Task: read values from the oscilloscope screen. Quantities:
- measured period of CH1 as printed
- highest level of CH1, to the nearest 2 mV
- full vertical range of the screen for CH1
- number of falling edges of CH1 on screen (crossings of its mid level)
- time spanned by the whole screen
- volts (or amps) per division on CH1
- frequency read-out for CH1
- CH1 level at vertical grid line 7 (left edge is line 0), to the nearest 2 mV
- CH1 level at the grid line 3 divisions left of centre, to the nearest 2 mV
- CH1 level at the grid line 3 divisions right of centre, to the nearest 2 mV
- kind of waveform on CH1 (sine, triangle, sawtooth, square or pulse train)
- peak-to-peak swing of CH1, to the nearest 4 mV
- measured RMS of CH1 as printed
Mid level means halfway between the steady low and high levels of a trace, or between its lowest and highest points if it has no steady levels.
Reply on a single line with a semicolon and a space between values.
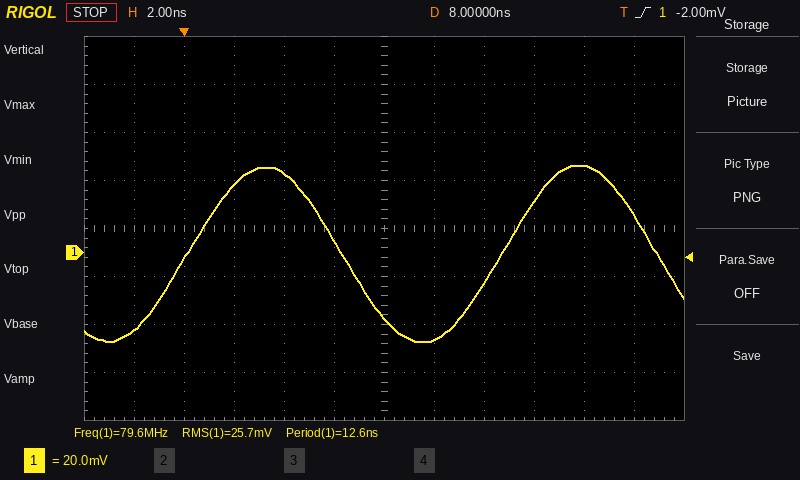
12.6 ns; 36 mV; 160 mV; 2; 24 ns; 20 mV; 79.6 MHz; -36 mV; 28 mV; 22 mV; sine; 72 mV; 25.7 mV
